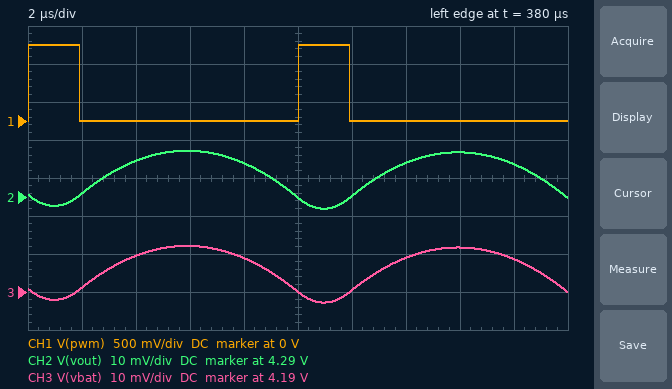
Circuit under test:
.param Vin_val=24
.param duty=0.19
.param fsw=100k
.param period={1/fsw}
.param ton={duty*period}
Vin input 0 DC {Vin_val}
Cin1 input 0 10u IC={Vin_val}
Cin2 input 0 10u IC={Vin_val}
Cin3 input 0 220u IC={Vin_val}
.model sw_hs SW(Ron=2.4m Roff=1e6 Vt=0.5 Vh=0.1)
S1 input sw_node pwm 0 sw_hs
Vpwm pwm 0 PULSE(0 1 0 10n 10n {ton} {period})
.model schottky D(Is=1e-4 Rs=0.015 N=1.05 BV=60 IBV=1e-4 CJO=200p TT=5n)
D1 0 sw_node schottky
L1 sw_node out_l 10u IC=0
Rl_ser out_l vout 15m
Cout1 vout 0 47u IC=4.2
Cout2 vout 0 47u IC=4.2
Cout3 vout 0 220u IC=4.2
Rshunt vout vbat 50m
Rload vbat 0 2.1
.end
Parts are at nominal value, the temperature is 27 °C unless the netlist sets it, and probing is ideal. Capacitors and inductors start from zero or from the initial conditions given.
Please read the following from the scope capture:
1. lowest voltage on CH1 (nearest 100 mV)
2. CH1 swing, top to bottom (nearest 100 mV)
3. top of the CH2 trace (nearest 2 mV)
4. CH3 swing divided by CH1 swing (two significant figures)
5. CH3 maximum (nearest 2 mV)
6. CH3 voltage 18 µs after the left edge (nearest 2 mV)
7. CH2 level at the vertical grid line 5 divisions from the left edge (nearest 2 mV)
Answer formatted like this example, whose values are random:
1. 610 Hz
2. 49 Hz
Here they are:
1. 0 V
2. 1.0 V
3. 4.302 V
4. 0.015
5. 4.202 V
6. 4.198 V
7. 4.290 V
